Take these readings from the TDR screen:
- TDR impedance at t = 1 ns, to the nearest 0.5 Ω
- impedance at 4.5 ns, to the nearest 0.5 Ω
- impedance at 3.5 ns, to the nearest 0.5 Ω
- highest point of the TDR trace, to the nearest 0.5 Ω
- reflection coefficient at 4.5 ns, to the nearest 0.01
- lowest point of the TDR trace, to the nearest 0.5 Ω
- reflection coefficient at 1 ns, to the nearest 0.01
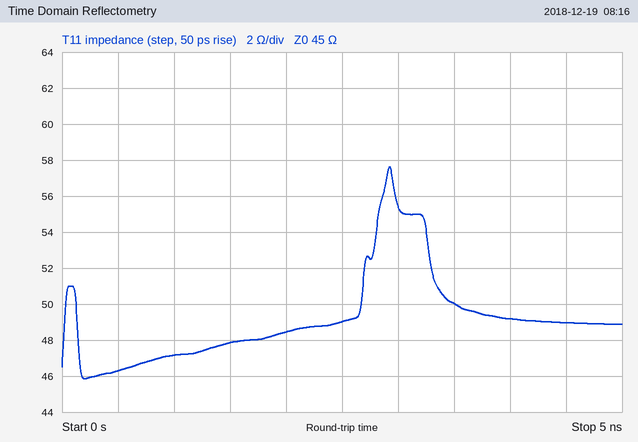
47.0 Ω
49.0 Ω
50.0 Ω
57.5 Ω
+0.04
46.0 Ω
+0.02
